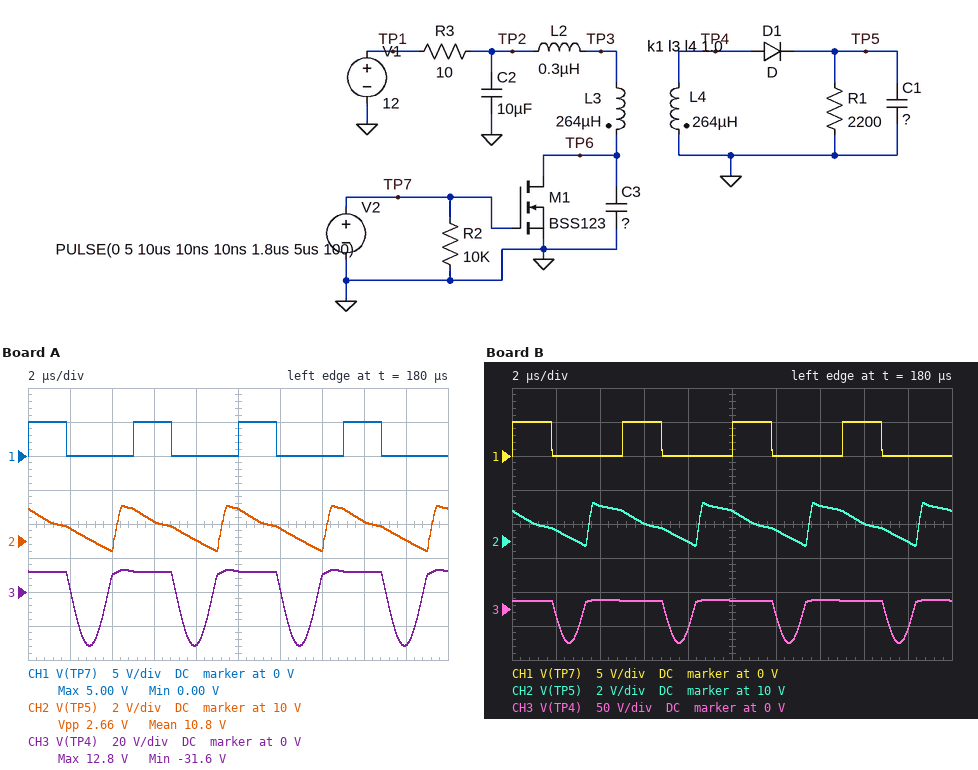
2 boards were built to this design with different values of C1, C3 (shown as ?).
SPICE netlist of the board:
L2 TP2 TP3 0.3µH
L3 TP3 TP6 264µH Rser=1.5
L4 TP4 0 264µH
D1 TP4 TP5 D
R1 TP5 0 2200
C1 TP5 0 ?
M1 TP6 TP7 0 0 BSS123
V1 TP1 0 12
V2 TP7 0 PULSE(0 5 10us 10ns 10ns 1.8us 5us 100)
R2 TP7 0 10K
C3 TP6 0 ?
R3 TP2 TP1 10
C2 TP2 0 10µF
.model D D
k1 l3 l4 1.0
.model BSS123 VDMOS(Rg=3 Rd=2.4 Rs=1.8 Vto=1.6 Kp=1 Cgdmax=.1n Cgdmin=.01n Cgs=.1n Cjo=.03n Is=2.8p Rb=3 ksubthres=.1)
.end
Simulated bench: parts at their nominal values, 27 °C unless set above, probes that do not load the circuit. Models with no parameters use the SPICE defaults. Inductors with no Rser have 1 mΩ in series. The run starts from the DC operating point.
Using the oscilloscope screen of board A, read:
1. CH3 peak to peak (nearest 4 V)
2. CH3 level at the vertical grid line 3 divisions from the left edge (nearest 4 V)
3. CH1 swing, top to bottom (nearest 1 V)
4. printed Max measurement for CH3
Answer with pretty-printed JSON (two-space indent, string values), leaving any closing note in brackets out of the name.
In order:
{
  "CH3 peak to peak": "44 V",
  "CH3 level at the vertical grid line 3 divisions from the left edge": "12 V",
  "CH1 swing, top to bottom": "5 V",
  "printed Max measurement for CH3": "12.8 V"
}
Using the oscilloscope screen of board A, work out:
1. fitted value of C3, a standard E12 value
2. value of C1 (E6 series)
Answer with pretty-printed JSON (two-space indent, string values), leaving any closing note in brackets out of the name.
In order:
{
  "fitted value of C3, a standard E12 value": "1.2 nF",
  "value of C1": "6.8 nF"
}
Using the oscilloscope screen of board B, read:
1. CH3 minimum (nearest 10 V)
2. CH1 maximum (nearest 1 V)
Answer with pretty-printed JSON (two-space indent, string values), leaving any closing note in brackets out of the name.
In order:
{
  "CH3 minimum": "-50 V",
  "CH1 maximum": "5 V"
}
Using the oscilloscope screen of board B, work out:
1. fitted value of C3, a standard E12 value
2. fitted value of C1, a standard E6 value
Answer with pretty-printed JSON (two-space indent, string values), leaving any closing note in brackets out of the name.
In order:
{
  "fitted value of C3, a standard E12 value": "680 pF",
  "fitted value of C1, a standard E6 value": "6.8 nF"
}
